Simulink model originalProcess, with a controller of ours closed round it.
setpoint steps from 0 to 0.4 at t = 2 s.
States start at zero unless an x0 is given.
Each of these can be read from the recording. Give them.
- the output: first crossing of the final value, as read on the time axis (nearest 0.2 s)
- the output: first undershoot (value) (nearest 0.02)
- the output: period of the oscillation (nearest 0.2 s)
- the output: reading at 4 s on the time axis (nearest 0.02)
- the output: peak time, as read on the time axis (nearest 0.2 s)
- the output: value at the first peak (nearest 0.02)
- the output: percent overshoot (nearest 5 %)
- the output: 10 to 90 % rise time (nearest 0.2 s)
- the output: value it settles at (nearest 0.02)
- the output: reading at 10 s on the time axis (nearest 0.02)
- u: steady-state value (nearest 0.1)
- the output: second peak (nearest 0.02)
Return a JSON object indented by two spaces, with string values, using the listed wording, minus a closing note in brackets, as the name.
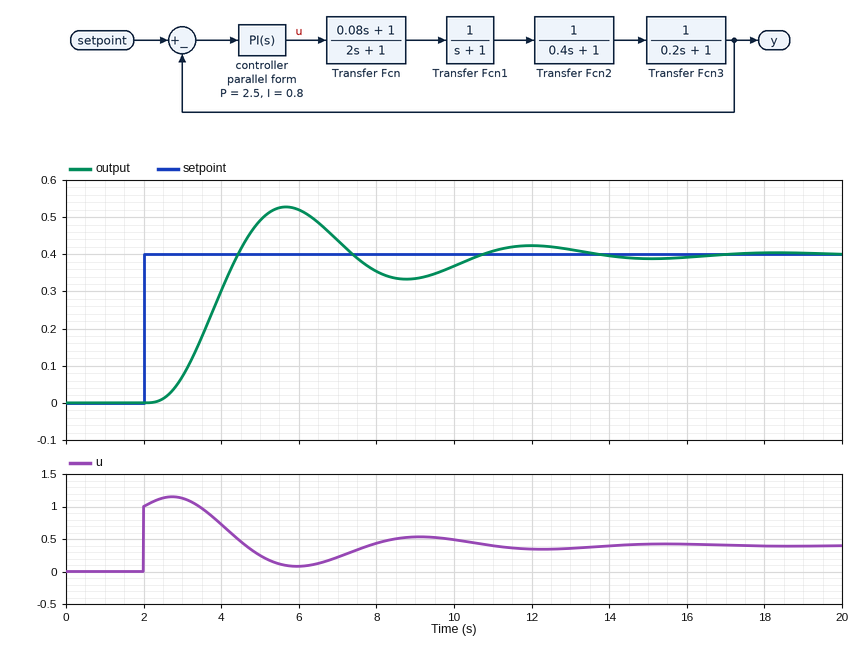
{
  "the output: first crossing of the final value, as read on the time axis": "4.4 s",
  "the output: first undershoot (value)": "0.34",
  "the output: period of the oscillation": "6.4 s",
  "the output: reading at 4 s on the time axis": "0.30",
  "the output: peak time, as read on the time axis": "5.6 s",
  "the output: value at the first peak": "0.52",
  "the output: percent overshoot": "30 %",
  "the output: 10 to 90 % rise time": "1.4 s",
  "the output: value it settles at": "0.40",
  "the output: reading at 10 s on the time axis": "0.36",
  "u: steady-state value": "0.4",
  "the output: second peak": "0.42"
}
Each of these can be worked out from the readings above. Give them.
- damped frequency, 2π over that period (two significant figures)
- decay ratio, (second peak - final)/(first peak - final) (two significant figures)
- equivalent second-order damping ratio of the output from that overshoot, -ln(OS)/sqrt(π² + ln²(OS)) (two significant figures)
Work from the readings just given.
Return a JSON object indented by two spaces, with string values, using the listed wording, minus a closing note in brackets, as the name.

{
  "damped frequency, 2π over that period": "0.98 rad/s",
  "decay ratio, (second peak - final)/(first peak - final)": "0.17",
  "equivalent second-order damping ratio of the output from that overshoot, -ln(OS)/sqrt(π² + ln²(OS))": "0.36"
}
